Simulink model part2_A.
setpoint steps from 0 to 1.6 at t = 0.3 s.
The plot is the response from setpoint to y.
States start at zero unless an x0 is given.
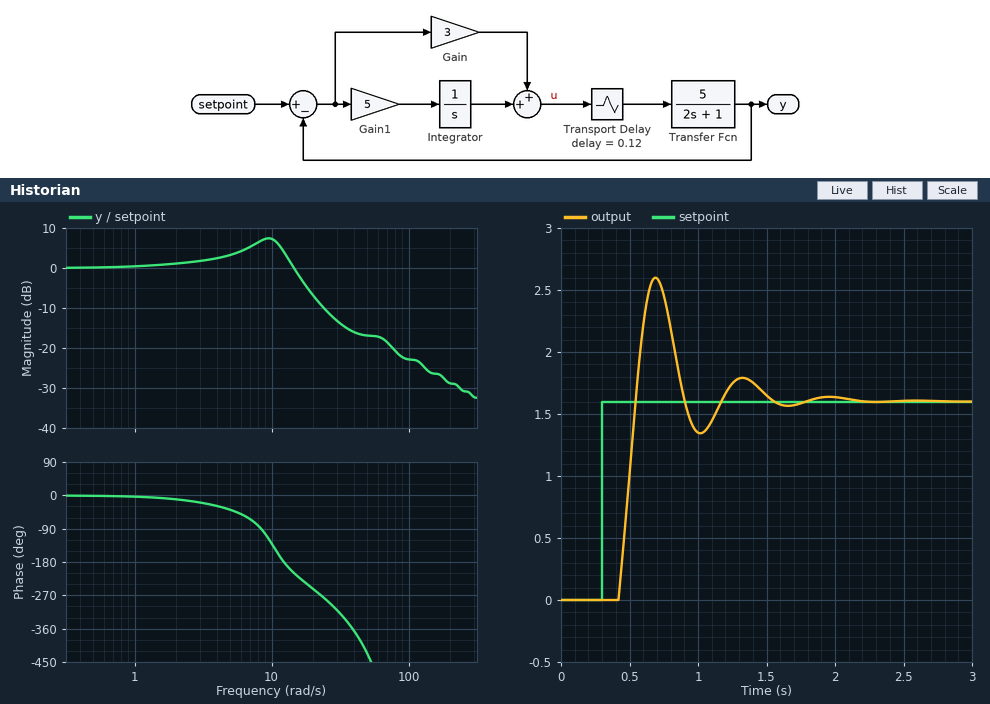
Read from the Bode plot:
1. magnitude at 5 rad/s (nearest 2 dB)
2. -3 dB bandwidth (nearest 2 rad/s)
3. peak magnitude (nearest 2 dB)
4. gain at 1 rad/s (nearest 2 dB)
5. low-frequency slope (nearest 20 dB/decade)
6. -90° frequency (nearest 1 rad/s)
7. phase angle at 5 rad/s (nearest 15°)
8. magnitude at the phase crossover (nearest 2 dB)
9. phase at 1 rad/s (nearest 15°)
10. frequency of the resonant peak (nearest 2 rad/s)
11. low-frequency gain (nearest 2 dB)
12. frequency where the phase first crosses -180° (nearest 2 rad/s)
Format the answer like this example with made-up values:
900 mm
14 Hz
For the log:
4 dB
16 rad/s
8 dB
0 dB
0 dB/decade
8 rad/s
-45°
4 dB
0°
10 rad/s
0 dB
12 rad/s
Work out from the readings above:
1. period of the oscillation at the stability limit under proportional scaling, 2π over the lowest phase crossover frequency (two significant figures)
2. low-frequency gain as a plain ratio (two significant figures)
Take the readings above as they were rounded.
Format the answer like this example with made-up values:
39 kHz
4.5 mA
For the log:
0.52 s
1.0
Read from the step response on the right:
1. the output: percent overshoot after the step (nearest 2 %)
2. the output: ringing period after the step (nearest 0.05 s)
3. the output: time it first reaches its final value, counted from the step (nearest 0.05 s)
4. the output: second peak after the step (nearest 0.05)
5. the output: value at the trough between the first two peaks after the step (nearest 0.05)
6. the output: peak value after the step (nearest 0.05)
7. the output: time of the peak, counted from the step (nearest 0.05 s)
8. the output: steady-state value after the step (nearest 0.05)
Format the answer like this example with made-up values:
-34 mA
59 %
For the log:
62 %
0.65 s
0.25 s
1.80
1.35
2.60
0.40 s
1.60
